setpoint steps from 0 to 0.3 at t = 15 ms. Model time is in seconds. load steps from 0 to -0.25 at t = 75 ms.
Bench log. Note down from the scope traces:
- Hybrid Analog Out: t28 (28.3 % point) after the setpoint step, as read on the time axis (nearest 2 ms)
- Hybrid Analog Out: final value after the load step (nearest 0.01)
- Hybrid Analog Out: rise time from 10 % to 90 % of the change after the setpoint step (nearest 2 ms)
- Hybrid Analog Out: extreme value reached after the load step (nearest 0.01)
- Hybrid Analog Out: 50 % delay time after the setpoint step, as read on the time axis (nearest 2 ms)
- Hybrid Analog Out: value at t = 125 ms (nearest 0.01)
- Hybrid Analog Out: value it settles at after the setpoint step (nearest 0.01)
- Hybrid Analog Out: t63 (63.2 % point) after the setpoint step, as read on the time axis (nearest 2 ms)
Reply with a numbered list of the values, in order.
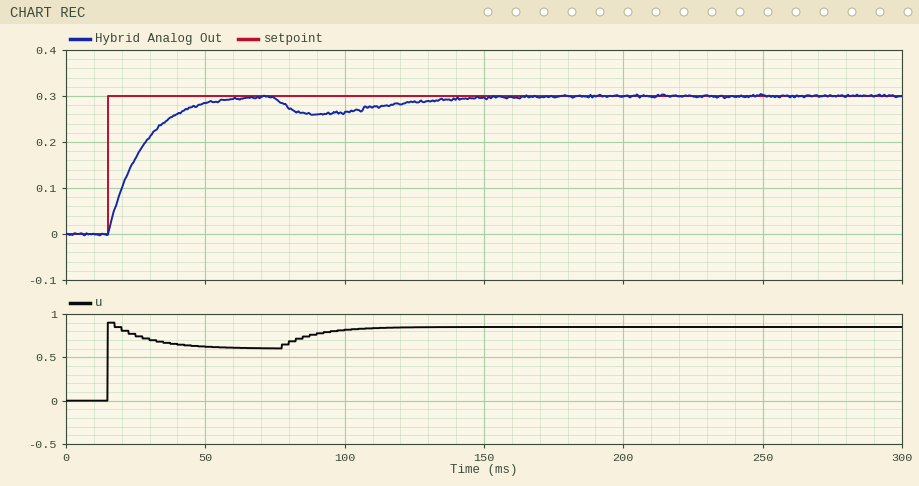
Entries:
1. 20 ms
2. 0.30
3. 26 ms
4. 0.26
5. 24 ms
6. 0.29
7. 0.30
8. 28 ms
